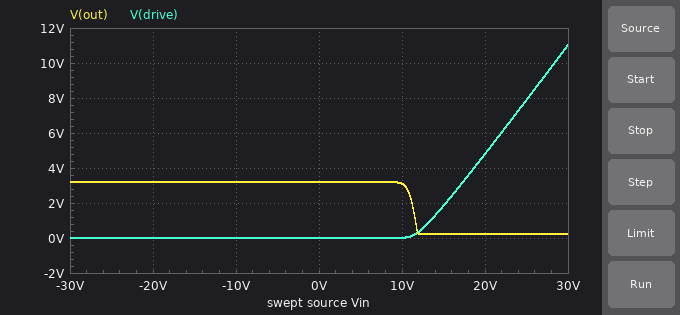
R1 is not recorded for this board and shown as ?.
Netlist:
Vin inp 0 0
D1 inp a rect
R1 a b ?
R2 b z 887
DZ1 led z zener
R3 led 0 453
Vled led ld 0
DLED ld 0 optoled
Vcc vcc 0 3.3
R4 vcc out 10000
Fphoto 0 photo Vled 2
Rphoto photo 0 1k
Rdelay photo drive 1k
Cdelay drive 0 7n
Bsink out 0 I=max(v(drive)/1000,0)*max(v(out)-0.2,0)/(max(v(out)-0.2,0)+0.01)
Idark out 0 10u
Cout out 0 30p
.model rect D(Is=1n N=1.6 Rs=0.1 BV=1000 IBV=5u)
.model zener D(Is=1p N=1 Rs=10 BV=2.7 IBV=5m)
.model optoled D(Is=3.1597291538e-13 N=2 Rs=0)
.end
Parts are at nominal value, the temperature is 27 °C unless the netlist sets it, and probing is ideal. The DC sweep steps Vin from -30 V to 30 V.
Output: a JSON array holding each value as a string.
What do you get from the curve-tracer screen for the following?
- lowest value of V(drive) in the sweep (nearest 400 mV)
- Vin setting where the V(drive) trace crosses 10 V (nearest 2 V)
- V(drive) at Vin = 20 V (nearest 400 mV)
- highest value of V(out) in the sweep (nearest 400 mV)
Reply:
["0 V", "28 V", "4.8 V", "3.2 V"]
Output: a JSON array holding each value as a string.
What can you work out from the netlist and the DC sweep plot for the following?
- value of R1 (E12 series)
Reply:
["2.2 kΩ"]
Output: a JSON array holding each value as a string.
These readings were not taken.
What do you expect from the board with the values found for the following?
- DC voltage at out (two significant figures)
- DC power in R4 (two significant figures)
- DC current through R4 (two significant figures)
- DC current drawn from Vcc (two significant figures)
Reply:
["3.2 V", "1.0 µW", "10 µA", "10 µA"]
